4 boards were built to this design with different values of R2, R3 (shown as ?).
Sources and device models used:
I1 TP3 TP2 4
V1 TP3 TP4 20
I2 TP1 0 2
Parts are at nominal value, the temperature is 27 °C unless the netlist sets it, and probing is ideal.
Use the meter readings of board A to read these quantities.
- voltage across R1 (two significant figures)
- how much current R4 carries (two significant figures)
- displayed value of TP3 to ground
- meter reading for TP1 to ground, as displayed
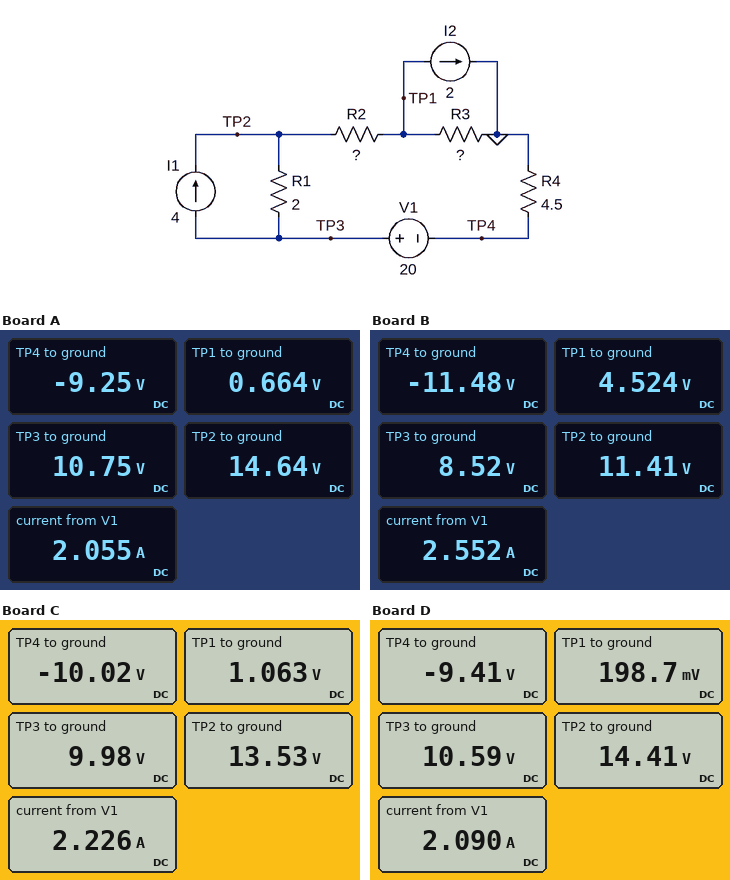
3.9 V
2.1 A
10.75 V
0.664 V
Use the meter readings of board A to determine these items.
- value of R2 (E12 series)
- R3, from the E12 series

6.8 Ω
12 Ω
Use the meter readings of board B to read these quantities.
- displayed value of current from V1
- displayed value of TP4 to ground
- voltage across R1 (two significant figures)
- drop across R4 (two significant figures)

2.552 A
-11.48 V
2.9 V
11 V
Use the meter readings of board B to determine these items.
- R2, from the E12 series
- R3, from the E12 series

2.7 Ω
8.2 Ω
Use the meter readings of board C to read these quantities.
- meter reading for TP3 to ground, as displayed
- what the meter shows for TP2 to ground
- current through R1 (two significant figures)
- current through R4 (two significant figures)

9.98 V
13.53 V
1.8 A
2.2 A
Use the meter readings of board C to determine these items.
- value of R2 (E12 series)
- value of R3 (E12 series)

5.6 Ω
4.7 Ω
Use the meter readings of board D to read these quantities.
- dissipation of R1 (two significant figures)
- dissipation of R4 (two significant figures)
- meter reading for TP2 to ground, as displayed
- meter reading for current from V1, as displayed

7.3 W
20 W
14.41 V
2.090 A
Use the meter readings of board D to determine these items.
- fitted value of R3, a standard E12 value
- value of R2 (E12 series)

2.2 Ω
6.8 Ω
